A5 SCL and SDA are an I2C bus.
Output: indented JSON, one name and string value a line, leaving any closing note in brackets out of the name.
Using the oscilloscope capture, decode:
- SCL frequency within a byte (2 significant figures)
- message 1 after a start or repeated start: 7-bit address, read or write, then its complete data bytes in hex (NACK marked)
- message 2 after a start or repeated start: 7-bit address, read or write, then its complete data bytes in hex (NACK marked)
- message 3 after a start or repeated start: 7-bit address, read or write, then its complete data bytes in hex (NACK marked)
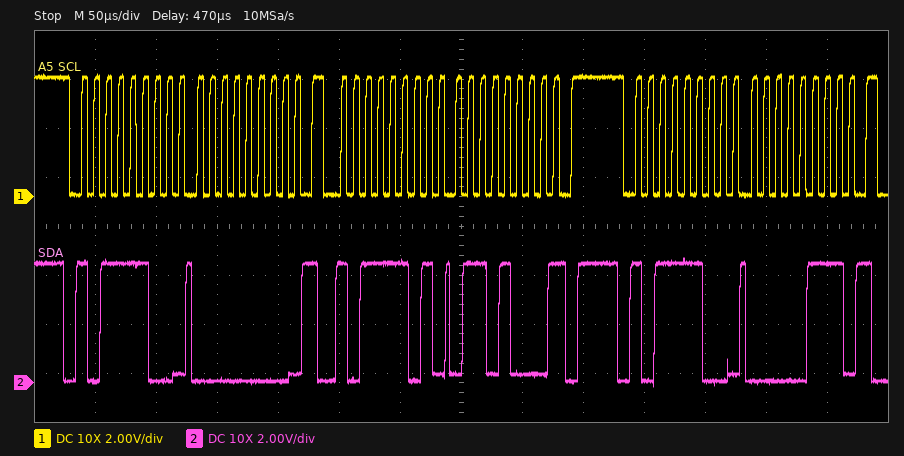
{
  "SCL frequency within a byte": "100 kHz",
  "message 1 after a start or repeated start: 7-bit address, read or write, then its complete data bytes in hex": "0x5E write: 00",
  "message 2 after a start or repeated start: 7-bit address, read or write, then its complete data bytes in hex": "0x5E read: 68 NACK",
  "message 3 after a start or repeated start: 7-bit address, read or write, then its complete data bytes in hex": "0x5E write: 07"
}
